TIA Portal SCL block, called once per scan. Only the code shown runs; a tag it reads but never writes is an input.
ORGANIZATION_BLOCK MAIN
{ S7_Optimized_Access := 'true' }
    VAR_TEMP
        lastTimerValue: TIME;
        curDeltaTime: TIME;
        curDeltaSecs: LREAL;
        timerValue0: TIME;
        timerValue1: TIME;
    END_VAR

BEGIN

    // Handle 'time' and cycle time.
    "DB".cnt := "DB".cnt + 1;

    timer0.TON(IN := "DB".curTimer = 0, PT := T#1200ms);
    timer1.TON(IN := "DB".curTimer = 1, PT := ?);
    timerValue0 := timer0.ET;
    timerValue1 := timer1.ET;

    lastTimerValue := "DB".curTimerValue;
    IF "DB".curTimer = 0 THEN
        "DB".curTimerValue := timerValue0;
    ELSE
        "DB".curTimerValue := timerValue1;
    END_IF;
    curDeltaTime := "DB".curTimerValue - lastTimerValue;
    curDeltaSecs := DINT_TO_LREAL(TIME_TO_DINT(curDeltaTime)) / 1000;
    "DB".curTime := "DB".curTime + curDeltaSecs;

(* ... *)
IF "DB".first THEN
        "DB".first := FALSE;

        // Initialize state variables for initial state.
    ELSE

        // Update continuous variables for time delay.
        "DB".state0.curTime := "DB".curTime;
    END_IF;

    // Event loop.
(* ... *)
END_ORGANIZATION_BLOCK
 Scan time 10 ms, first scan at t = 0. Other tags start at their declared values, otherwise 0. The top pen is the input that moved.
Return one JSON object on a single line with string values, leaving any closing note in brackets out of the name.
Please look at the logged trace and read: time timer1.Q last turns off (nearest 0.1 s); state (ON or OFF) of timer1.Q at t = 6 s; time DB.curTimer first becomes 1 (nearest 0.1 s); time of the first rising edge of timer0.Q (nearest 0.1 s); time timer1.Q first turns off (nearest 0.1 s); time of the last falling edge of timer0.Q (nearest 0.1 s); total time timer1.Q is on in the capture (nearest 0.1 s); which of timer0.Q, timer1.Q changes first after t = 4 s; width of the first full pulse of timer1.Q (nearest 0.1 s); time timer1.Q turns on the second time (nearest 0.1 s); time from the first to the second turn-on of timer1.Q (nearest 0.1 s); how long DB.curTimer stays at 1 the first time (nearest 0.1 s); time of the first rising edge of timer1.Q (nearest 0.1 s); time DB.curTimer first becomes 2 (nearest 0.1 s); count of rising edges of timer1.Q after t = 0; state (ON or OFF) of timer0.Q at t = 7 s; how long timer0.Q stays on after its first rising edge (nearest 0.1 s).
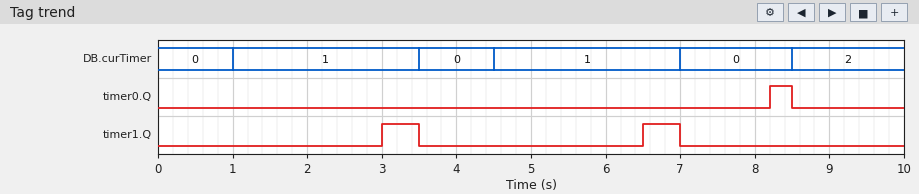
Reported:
{"time timer1.Q last turns off": "7.0 s", "state (ON or OFF) of timer1.Q at t = 6 s": "OFF", "time DB.curTimer first becomes 1": "1.0 s", "time of the first rising edge of timer0.Q": "8.2 s", "time timer1.Q first turns off": "3.5 s", "time of the last falling edge of timer0.Q": "8.5 s", "total time timer1.Q is on in the capture": "1.0 s", "which of timer0.Q, timer1.Q changes first after t = 4 s": "timer1.Q", "width of the first full pulse of timer1.Q": "0.5 s", "time timer1.Q turns on the second time": "6.5 s", "time from the first to the second turn-on of timer1.Q": "3.5 s", "how long DB.curTimer stays at 1 the first time": "2.5 s", "time of the first rising edge of timer1.Q": "3.0 s", "time DB.curTimer first becomes 2": "8.5 s", "count of rising edges of timer1.Q after t = 0": "2", "state (ON or OFF) of timer0.Q at t = 7 s": "OFF", "how long timer0.Q stays on after its first rising edge": "0.3 s"}
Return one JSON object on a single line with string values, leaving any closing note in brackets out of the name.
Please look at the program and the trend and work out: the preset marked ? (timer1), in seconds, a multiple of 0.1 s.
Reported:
{"the preset marked ? (timer1), in seconds, a multiple of 0.1 s": "2.0 s"}
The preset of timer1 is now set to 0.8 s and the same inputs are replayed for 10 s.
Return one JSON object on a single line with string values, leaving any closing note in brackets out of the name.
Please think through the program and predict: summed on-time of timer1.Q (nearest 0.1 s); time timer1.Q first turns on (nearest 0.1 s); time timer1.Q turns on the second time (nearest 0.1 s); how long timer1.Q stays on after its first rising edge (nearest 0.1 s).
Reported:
{"summed on-time of timer1.Q": "3.4 s", "time timer1.Q first turns on": "1.8 s", "time timer1.Q turns on the second time": "5.3 s", "how long timer1.Q stays on after its first rising edge": "1.7 s"}
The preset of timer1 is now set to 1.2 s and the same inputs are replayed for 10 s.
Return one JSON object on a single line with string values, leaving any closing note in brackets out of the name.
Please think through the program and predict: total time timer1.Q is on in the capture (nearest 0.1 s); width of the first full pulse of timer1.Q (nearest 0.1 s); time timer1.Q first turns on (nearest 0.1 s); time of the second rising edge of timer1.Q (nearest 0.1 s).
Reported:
{"total time timer1.Q is on in the capture": "2.6 s", "width of the first full pulse of timer1.Q": "1.3 s", "time timer1.Q first turns on": "2.2 s", "time of the second rising edge of timer1.Q": "5.7 s"}
